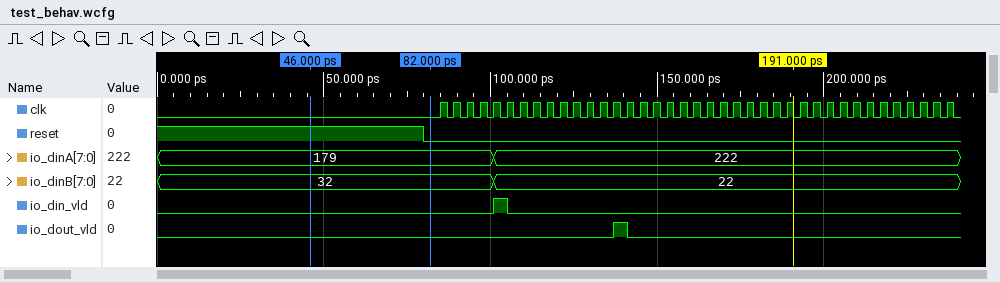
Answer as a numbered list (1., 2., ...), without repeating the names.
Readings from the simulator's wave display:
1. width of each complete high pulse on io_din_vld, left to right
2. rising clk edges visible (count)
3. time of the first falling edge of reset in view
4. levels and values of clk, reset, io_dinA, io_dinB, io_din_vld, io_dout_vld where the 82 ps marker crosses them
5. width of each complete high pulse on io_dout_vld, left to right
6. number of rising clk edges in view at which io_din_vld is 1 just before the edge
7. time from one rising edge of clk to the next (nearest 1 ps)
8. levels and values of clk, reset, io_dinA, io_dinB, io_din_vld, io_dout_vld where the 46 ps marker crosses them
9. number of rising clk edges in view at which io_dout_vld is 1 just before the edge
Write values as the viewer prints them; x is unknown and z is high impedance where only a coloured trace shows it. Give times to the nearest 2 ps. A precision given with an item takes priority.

1. 4 ps
2. 39
3. 80 ps
4. clk=0, reset=0, io_dinA=179, io_dinB=32, io_din_vld=0, io_dout_vld=0
5. 4 ps
6. 1
7. 4 ps
8. clk=0, reset=1, io_dinA=179, io_dinB=32, io_din_vld=0, io_dout_vld=0
9. 1
